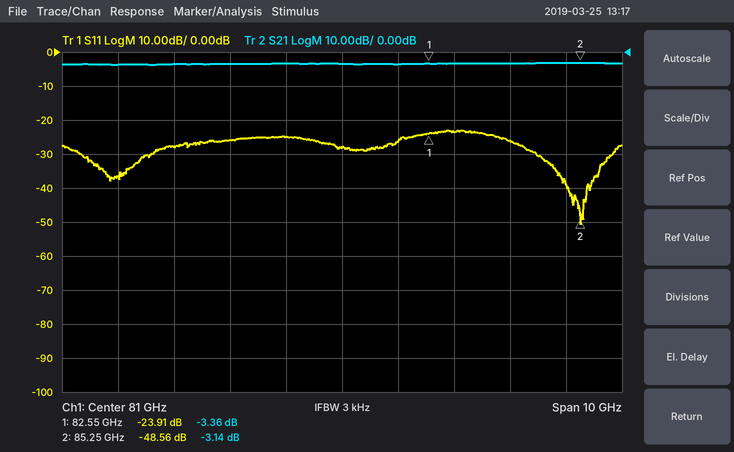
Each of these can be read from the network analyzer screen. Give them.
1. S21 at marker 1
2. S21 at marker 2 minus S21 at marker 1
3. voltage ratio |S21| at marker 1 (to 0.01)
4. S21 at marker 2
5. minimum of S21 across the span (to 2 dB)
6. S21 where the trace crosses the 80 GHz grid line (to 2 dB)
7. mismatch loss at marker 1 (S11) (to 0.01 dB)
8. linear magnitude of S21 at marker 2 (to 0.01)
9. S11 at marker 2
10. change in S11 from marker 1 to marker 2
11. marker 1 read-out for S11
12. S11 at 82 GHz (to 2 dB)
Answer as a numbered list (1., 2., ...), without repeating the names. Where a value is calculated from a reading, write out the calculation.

1. -3.36 dB
2. -3.14 − (-3.36) = 0.22 dB
3. 10^(-3.36/20) ≈ 0.68
4. -3.14 dB
5. -4 dB
6. -4 dB
7. −10 log10(1 − 10^(-23.91/10)) ≈ 0.02 dB
8. 10^(-3.14/20) ≈ 0.70
9. -48.56 dB
10. -48.56 − (-23.91) = -24.65 dB
11. -23.91 dB
12. -26 dB
